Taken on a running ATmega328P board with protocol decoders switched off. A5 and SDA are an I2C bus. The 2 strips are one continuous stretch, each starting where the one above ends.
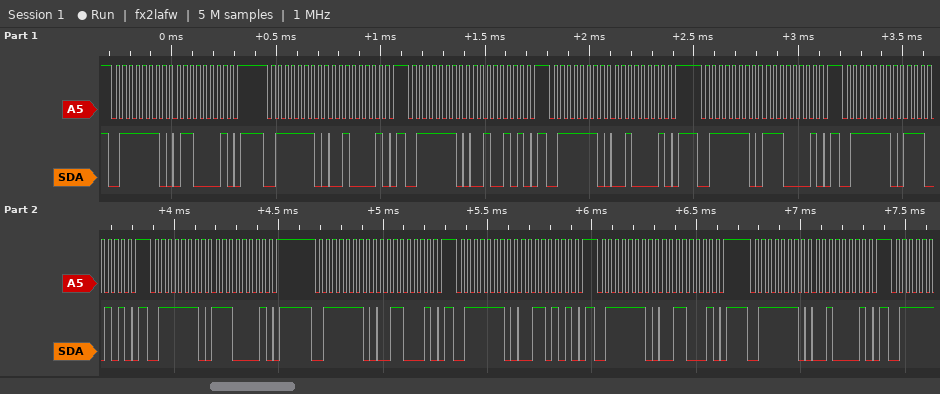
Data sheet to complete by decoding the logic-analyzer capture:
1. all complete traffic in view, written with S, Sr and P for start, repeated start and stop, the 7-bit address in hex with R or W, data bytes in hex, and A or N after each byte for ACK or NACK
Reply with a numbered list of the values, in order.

1. S 3FW A 61 A P S 3FW A 21 A P S 3FW A 25 A P S 3FW A 21 A P S 3FW A E1 A P S 3FW A E5 A P S 3FW A E1 A P S 3FW A 31 A P S 3FW A 35 A P S 3FW A 31 A P S 3FW A 21 A P
